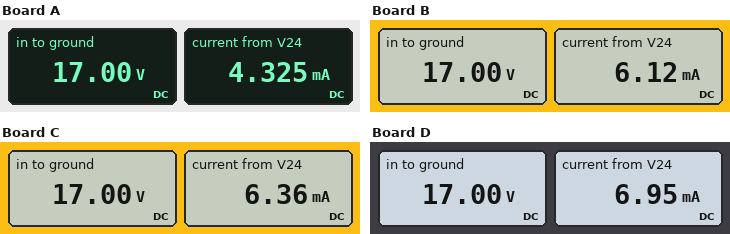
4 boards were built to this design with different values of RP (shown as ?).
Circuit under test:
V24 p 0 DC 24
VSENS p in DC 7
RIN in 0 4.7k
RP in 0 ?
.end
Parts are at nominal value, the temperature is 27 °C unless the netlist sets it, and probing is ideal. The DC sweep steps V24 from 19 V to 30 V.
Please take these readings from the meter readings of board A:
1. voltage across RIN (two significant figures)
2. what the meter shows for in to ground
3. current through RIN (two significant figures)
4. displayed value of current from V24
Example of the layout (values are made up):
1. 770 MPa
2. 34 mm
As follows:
1. 17 V
2. 17.00 V
3. 3.6 mA
4. 4.325 mA
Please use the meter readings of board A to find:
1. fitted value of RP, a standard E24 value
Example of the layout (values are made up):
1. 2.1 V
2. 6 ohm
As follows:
1. 24 kΩ
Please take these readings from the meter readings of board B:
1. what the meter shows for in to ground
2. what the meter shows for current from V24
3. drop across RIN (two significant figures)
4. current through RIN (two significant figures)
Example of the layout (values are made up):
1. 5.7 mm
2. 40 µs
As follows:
1. 17.00 V
2. 6.12 mA
3. 17 V
4. 3.6 mA
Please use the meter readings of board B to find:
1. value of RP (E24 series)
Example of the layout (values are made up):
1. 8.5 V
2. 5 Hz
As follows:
1. 6.8 kΩ
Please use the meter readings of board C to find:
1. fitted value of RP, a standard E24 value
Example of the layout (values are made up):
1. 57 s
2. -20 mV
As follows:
1. 6.2 kΩ
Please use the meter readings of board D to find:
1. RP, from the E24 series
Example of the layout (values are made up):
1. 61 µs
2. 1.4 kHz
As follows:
1. 5.1 kΩ
